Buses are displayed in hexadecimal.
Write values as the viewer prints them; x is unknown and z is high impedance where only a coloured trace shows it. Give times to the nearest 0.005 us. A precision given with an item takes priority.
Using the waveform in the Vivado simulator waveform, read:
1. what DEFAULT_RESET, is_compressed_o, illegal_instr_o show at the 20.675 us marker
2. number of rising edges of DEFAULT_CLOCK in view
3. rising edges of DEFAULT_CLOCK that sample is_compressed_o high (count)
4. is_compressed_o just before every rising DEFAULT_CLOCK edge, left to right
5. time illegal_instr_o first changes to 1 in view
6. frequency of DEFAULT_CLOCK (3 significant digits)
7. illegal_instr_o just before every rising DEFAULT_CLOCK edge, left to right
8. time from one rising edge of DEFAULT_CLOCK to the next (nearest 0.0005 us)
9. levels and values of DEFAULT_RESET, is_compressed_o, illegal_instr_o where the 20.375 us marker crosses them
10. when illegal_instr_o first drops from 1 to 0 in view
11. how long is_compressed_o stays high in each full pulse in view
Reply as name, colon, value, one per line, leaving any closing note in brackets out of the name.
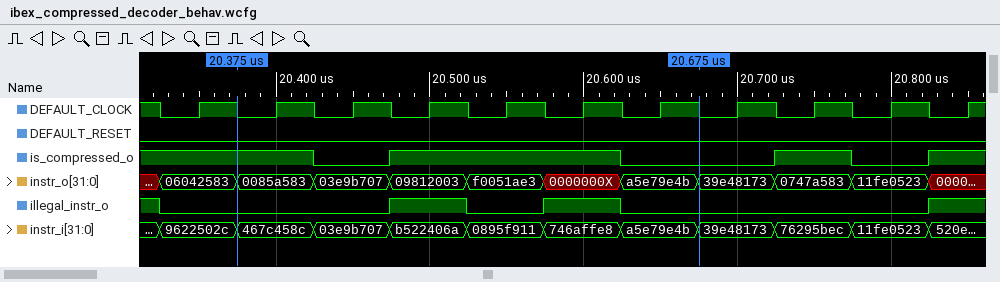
what DEFAULT_RESET, is_compressed_o, illegal_instr_o show at the 20.675 us marker: DEFAULT_RESET=0, is_compressed_o=0, illegal_instr_o=0
number of rising edges of DEFAULT_CLOCK in view: 11
rising edges of DEFAULT_CLOCK that sample is_compressed_o high: 7
is_compressed_o just before every rising DEFAULT_CLOCK edge, left to right: 1 1 0 1 1 1 0 0 1 0 1
time illegal_instr_o first changes to 1 in view: 20.475 us
frequency of DEFAULT_CLOCK: 20.0 MHz
illegal_instr_o just before every rising DEFAULT_CLOCK edge, left to right: 0 0 0 1 0 1 0 0 0 0 1
time from one rising edge of DEFAULT_CLOCK to the next: 0.05 us
levels and values of DEFAULT_RESET, is_compressed_o, illegal_instr_o where the 20.375 us marker crosses them: DEFAULT_RESET=0, is_compressed_o=1, illegal_instr_o=0
when illegal_instr_o first drops from 1 to 0 in view: 20.325 us
how long is_compressed_o stays high in each full pulse in view: 0.15 us, 0.05 us
